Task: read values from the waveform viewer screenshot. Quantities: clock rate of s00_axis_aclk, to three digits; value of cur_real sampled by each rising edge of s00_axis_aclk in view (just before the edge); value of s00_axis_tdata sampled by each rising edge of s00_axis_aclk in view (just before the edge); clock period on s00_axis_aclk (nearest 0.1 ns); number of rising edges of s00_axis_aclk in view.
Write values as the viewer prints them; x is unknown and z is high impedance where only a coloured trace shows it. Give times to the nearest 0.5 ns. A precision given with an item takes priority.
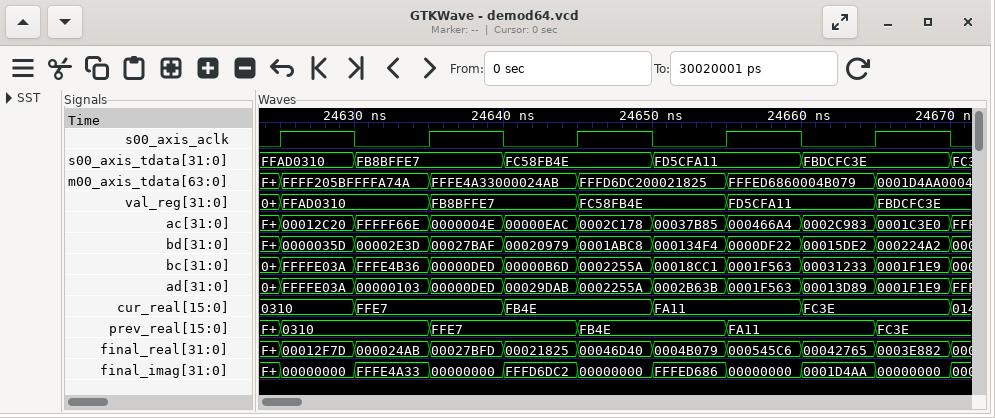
100 MHz
0310, FFE7, FB4E, FA11, FC3E
FFAD0310, FB8BFFE7, FC58FB4E, FD5CFA11, FBDCFC3E
10 ns
5
